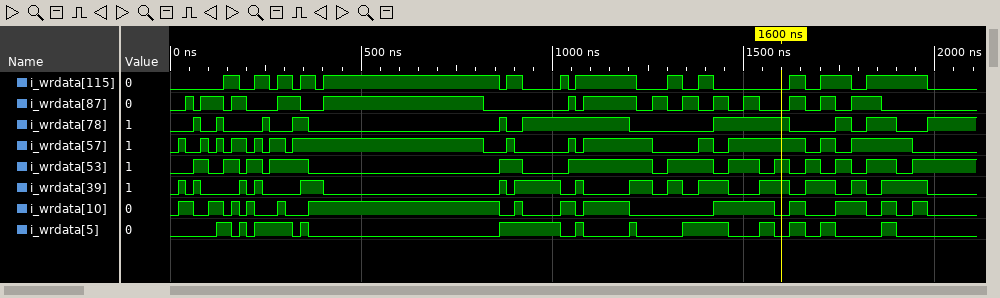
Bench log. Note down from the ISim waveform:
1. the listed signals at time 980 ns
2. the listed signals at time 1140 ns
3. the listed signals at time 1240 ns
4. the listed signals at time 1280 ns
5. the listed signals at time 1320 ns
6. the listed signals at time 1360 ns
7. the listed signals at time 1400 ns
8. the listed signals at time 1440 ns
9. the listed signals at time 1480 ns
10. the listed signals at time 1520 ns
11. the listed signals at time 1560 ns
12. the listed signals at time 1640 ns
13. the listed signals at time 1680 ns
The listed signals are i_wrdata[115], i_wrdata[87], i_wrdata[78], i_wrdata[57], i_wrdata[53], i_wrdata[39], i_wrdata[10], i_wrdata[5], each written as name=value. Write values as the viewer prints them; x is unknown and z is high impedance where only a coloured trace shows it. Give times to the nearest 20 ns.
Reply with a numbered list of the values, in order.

1. i_wrdata[115]=0, i_wrdata[87]=0, i_wrdata[78]=1, i_wrdata[57]=0, i_wrdata[53]=0, i_wrdata[39]=1, i_wrdata[10]=0, i_wrdata[5]=1
2. i_wrdata[115]=1, i_wrdata[87]=1, i_wrdata[78]=1, i_wrdata[57]=1, i_wrdata[53]=1, i_wrdata[39]=0, i_wrdata[10]=1, i_wrdata[5]=0
3. i_wrdata[115]=0, i_wrdata[87]=0, i_wrdata[78]=0, i_wrdata[57]=1, i_wrdata[53]=1, i_wrdata[39]=1, i_wrdata[10]=0, i_wrdata[5]=0
4. i_wrdata[115]=0, i_wrdata[87]=1, i_wrdata[78]=0, i_wrdata[57]=0, i_wrdata[53]=0, i_wrdata[39]=0, i_wrdata[10]=0, i_wrdata[5]=0
5. i_wrdata[115]=1, i_wrdata[87]=0, i_wrdata[78]=0, i_wrdata[57]=0, i_wrdata[53]=1, i_wrdata[39]=1, i_wrdata[10]=0, i_wrdata[5]=0
6. i_wrdata[115]=0, i_wrdata[87]=1, i_wrdata[78]=0, i_wrdata[57]=0, i_wrdata[53]=1, i_wrdata[39]=0, i_wrdata[10]=0, i_wrdata[5]=1
7. i_wrdata[115]=1, i_wrdata[87]=0, i_wrdata[78]=0, i_wrdata[57]=1, i_wrdata[53]=1, i_wrdata[39]=1, i_wrdata[10]=0, i_wrdata[5]=1
8. i_wrdata[115]=0, i_wrdata[87]=1, i_wrdata[78]=1, i_wrdata[57]=0, i_wrdata[53]=0, i_wrdata[39]=1, i_wrdata[10]=1, i_wrdata[5]=1
9. i_wrdata[115]=0, i_wrdata[87]=0, i_wrdata[78]=1, i_wrdata[57]=1, i_wrdata[53]=1, i_wrdata[39]=0, i_wrdata[10]=1, i_wrdata[5]=0
10. i_wrdata[115]=0, i_wrdata[87]=1, i_wrdata[78]=1, i_wrdata[57]=1, i_wrdata[53]=1, i_wrdata[39]=0, i_wrdata[10]=1, i_wrdata[5]=0
11. i_wrdata[115]=0, i_wrdata[87]=0, i_wrdata[78]=1, i_wrdata[57]=1, i_wrdata[53]=0, i_wrdata[39]=1, i_wrdata[10]=1, i_wrdata[5]=1
12. i_wrdata[115]=1, i_wrdata[87]=1, i_wrdata[78]=0, i_wrdata[57]=1, i_wrdata[53]=0, i_wrdata[39]=0, i_wrdata[10]=1, i_wrdata[5]=1
13. i_wrdata[115]=0, i_wrdata[87]=0, i_wrdata[78]=0, i_wrdata[57]=0, i_wrdata[53]=1, i_wrdata[39]=1, i_wrdata[10]=0, i_wrdata[5]=0
